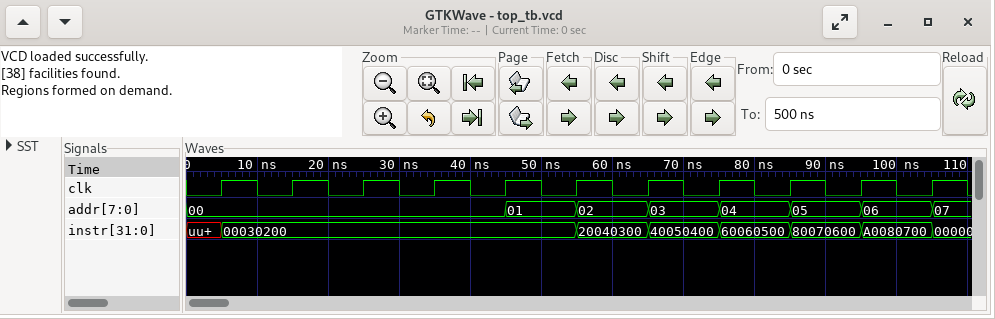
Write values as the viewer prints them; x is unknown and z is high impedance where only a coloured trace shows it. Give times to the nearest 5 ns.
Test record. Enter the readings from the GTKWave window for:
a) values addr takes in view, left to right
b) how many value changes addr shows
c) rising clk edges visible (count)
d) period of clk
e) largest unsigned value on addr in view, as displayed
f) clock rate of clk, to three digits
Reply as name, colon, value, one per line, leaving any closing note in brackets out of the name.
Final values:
values addr takes in view, left to right: 00, 01, 02, 03, 04, 05, 06, 07
how many value changes addr shows: 7
rising clk edges visible: 11
period of clk: 10 ns
largest unsigned value on addr in view, as displayed: 07
clock rate of clk, to three digits: 100 MHz
